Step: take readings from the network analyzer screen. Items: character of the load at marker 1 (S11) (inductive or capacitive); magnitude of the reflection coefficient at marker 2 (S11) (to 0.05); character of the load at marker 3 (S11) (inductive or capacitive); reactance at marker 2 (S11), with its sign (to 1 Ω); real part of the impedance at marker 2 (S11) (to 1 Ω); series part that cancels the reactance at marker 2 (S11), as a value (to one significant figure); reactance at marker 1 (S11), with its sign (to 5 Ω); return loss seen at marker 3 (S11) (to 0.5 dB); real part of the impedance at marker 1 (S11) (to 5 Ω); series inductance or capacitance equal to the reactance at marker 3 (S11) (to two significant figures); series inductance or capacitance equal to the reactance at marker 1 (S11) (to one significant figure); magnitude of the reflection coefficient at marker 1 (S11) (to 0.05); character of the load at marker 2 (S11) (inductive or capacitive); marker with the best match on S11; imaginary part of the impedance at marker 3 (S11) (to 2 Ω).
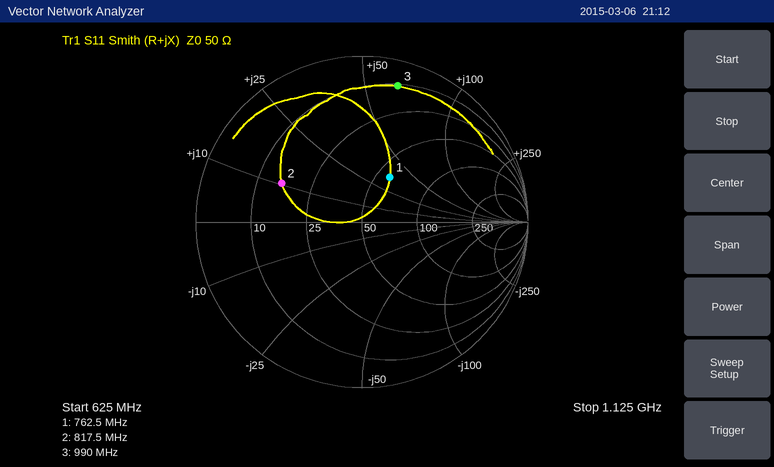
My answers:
inductive
0.55
inductive
+10 Ω
16 Ω
20 pF
+35 Ω
1.5 dB
60 Ω
10 nH
7 nH
0.30
inductive
marker 1
+64 Ω
